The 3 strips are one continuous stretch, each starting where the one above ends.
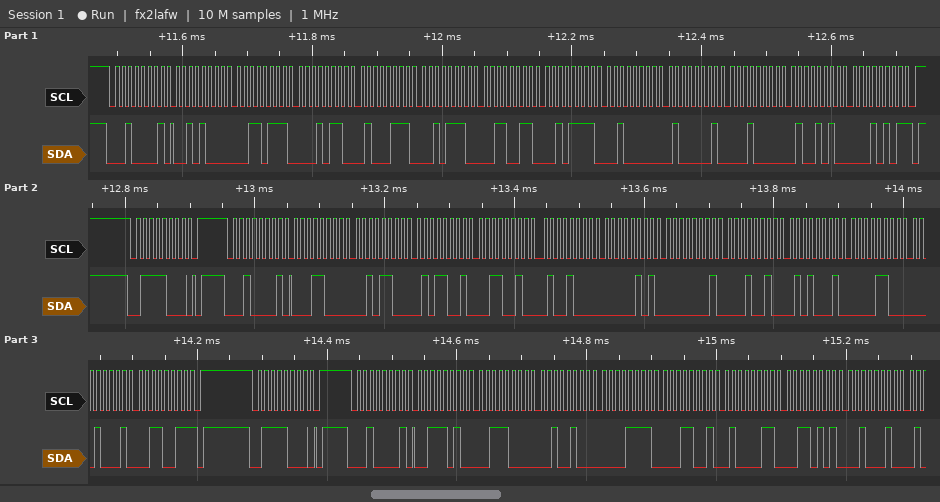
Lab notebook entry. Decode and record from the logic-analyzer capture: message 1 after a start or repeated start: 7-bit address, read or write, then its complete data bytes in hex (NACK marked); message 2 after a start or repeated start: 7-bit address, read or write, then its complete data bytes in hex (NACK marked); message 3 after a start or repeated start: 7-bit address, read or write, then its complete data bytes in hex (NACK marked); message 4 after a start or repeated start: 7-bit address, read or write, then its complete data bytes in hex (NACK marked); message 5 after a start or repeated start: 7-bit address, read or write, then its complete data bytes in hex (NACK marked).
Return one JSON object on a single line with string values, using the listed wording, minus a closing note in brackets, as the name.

{"message 1 after a start or repeated start: 7-bit address, read or write, then its complete data bytes in hex": "0x10 read: 28 37 16 47 2E 33 2F 20 41 10 4A 15 NACK", "message 2 after a start or repeated start: 7-bit address, read or write, then its complete data bytes in hex": "0x3C write", "message 3 after a start or repeated start: 7-bit address, read or write, then its complete data bytes in hex": "0x10 read: 18 2C 59 32 48 05 01 12 51 0C 11 33 NACK", "message 4 after a start or repeated start: 7-bit address, read or write, then its complete data bytes in hex": "0x3C write", "message 5 after a start or repeated start: 7-bit address, read or write, then its complete data bytes in hex": "0x10 read: 3A 38 24 0F 19 43 35 22"}
